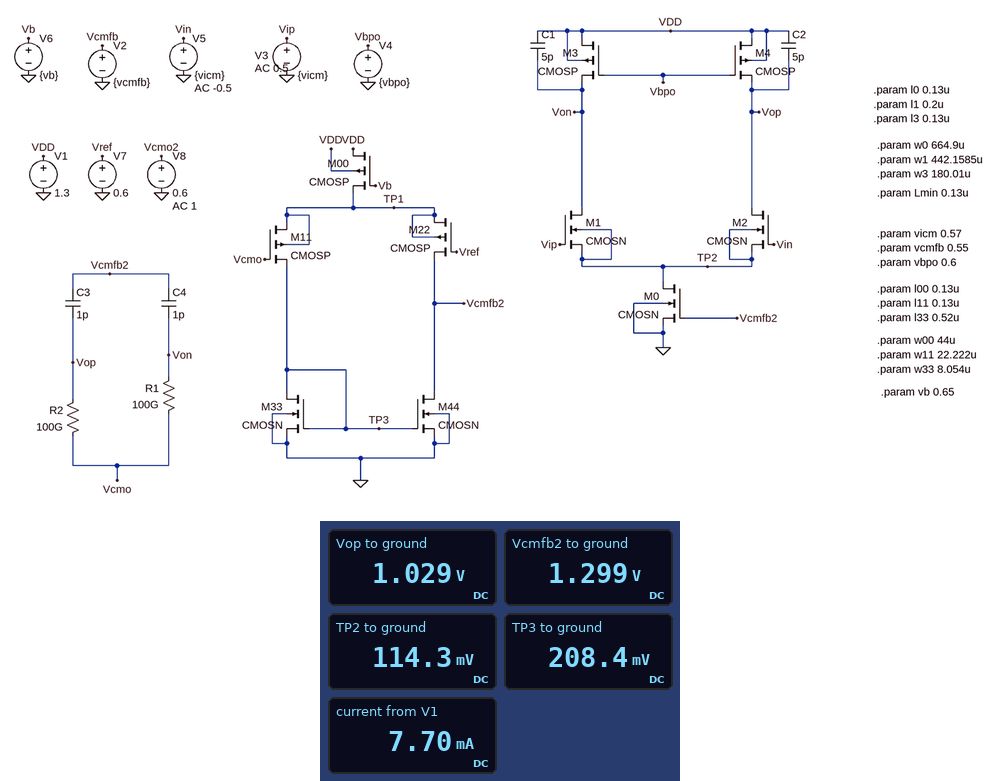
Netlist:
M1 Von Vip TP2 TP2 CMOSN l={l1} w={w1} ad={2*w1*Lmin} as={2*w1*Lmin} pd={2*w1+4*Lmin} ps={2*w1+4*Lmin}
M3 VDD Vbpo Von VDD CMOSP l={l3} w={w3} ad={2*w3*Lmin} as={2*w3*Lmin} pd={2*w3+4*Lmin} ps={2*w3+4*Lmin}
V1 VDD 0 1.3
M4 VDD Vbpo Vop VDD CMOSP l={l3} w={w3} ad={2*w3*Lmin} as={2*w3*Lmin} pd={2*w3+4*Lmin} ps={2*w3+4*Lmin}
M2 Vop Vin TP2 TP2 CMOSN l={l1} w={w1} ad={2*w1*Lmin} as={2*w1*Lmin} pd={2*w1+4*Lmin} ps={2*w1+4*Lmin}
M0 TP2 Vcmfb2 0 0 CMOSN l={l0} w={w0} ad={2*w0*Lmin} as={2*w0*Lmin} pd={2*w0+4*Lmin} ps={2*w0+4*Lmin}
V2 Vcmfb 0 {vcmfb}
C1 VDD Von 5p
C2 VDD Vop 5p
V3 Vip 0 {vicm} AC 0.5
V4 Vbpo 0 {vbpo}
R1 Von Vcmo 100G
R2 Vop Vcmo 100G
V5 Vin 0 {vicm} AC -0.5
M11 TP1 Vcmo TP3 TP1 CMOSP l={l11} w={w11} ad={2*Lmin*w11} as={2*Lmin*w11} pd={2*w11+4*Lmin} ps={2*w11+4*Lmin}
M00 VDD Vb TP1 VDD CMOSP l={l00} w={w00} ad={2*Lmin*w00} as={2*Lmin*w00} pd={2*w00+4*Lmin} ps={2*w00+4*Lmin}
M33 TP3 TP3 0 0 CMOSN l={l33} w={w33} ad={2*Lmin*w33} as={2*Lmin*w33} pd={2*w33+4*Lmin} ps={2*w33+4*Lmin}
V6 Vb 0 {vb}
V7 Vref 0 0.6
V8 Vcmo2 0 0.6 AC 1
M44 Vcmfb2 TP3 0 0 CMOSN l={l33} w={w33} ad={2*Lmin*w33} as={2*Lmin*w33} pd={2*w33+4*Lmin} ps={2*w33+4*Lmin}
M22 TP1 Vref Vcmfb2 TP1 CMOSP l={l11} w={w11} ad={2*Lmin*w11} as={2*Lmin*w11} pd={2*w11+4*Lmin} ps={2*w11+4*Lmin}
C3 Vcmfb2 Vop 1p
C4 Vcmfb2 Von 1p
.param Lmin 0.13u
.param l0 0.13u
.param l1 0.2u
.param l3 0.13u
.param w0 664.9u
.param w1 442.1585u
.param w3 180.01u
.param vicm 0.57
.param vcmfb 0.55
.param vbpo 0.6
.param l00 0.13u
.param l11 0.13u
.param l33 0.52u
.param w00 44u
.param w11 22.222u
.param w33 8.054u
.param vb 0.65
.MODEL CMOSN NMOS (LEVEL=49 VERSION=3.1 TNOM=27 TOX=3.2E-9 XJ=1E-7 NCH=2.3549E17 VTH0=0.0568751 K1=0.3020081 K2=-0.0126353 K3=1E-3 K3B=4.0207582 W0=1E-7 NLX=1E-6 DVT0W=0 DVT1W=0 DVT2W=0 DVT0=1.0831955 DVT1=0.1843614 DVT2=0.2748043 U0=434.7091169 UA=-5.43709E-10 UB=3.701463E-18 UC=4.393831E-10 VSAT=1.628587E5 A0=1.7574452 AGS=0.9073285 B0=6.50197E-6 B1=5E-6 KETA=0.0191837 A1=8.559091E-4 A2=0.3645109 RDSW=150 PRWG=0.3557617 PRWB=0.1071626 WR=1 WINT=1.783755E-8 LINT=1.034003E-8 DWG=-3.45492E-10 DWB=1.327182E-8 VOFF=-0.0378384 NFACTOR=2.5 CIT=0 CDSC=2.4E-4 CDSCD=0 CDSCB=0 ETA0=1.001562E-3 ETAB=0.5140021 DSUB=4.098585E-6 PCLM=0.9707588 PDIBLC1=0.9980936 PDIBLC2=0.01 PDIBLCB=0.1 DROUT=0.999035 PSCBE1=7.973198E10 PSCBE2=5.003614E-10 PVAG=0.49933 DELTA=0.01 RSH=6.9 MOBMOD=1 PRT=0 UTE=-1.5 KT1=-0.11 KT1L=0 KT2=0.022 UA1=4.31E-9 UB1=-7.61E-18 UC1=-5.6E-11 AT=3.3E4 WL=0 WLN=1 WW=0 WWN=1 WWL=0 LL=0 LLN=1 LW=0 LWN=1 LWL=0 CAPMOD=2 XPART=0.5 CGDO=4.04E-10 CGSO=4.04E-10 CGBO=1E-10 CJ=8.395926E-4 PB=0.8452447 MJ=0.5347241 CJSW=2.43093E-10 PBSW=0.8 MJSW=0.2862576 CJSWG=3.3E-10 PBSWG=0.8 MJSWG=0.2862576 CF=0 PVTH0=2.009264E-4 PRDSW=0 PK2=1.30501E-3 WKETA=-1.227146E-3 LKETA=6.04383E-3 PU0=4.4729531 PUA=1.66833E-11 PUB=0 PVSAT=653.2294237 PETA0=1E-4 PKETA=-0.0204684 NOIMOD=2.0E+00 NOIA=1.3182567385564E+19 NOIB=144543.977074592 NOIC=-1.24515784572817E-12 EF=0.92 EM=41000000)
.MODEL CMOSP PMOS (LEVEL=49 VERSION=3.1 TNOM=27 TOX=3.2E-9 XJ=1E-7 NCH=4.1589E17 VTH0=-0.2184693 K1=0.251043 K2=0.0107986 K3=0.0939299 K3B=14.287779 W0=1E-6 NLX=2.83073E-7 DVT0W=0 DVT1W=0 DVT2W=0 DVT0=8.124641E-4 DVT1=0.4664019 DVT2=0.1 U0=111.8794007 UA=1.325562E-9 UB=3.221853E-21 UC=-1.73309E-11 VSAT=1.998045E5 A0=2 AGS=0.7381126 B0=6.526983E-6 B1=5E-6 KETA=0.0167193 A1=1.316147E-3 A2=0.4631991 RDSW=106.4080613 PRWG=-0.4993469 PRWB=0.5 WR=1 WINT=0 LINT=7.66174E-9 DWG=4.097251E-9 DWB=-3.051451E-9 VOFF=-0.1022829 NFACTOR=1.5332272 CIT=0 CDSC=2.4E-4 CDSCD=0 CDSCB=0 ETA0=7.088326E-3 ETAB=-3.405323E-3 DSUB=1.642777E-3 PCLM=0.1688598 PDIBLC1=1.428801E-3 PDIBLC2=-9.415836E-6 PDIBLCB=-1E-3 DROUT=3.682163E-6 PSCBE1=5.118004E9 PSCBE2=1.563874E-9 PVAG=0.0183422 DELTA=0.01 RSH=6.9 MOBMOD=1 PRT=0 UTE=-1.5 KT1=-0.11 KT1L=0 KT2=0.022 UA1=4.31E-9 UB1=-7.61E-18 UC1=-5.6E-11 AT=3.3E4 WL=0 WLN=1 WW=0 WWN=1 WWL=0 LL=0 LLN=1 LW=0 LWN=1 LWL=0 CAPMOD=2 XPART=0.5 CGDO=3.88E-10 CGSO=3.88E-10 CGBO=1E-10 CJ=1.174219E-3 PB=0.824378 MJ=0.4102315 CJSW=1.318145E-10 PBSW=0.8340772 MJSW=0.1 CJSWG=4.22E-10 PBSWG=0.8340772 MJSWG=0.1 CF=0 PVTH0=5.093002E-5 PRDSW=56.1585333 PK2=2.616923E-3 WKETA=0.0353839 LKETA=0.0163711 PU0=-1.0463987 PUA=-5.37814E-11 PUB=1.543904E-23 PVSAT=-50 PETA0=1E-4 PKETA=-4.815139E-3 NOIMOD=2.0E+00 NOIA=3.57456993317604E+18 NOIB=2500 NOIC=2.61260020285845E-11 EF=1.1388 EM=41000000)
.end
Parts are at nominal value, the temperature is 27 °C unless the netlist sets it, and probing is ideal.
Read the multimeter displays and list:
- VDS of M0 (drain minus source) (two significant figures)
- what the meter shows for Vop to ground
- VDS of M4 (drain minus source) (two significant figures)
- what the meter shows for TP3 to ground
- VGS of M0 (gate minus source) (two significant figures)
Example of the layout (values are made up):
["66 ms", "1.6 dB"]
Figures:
["110 mV", "1.029 V", "270 mV", "208.4 mV", "1.3 V"]
